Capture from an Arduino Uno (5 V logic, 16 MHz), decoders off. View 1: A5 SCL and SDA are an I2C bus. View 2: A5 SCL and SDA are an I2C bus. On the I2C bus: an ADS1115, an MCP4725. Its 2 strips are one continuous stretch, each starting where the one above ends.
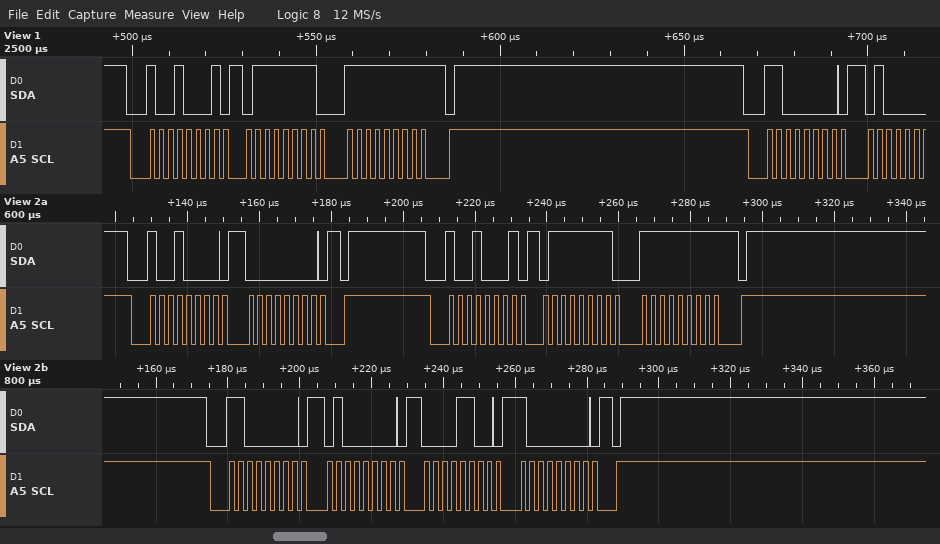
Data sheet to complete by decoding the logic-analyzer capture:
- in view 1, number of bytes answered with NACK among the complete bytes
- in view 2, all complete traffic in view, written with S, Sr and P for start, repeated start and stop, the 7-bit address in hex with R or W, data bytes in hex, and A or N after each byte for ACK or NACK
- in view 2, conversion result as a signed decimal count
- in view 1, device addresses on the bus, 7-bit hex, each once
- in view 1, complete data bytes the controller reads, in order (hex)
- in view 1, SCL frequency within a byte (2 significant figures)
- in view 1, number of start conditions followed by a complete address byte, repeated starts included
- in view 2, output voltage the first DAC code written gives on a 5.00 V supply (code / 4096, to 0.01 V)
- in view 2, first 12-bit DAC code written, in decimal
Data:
1
S 48W A 00 A P S 48R A 7F A FF N P S 60W A 40 A 0C A 80 A P
32767
0x48 0x60
7F FF
400 kHz
2
0.24 V
200
